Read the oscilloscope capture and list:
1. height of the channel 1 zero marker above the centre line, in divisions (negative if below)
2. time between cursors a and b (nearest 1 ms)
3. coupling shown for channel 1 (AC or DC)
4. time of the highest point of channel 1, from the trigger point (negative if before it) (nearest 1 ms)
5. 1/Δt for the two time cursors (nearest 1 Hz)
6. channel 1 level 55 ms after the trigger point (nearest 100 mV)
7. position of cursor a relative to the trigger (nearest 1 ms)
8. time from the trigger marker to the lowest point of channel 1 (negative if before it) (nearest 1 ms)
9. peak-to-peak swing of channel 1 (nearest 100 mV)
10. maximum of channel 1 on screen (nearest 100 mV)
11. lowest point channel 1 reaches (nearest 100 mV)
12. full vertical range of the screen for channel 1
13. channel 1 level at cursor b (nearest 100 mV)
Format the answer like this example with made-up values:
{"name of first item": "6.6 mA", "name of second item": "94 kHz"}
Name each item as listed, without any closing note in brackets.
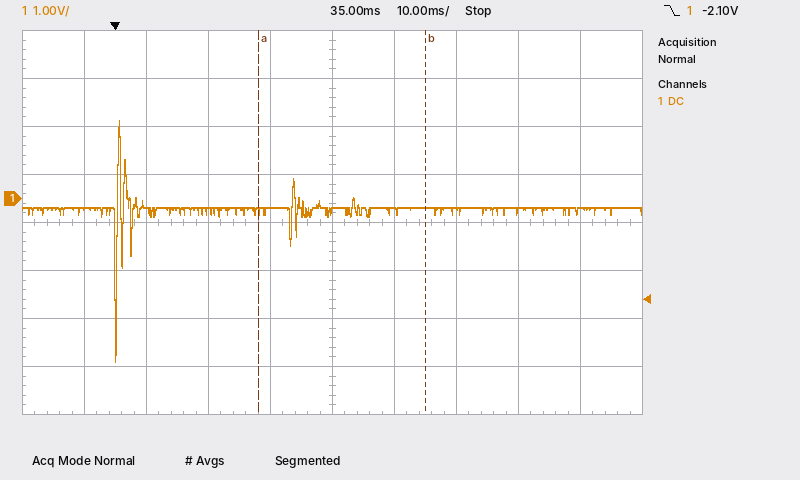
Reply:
{"height of the channel 1 zero marker above the centre line, in divisions": "+0.5 div", "time between cursors a and b": "27 ms", "coupling shown for channel 1": "DC", "time of the highest point of channel 1, from the trigger point (negative if before it)": "+1 ms", "1/Δt for the two time cursors": "37 Hz", "channel 1 level 55 ms after the trigger point": "-200 mV", "position of cursor a relative to the trigger": "+23 ms", "time from the trigger marker to the lowest point of channel 1 (negative if before it)": "0 ms", "peak-to-peak swing of channel 1": "5.0 V", "maximum of channel 1 on screen": "1.6 V", "lowest point channel 1 reaches": "-3.4 V", "full vertical range of the screen for channel 1": "8 V", "channel 1 level at cursor b": "-200 mV"}
